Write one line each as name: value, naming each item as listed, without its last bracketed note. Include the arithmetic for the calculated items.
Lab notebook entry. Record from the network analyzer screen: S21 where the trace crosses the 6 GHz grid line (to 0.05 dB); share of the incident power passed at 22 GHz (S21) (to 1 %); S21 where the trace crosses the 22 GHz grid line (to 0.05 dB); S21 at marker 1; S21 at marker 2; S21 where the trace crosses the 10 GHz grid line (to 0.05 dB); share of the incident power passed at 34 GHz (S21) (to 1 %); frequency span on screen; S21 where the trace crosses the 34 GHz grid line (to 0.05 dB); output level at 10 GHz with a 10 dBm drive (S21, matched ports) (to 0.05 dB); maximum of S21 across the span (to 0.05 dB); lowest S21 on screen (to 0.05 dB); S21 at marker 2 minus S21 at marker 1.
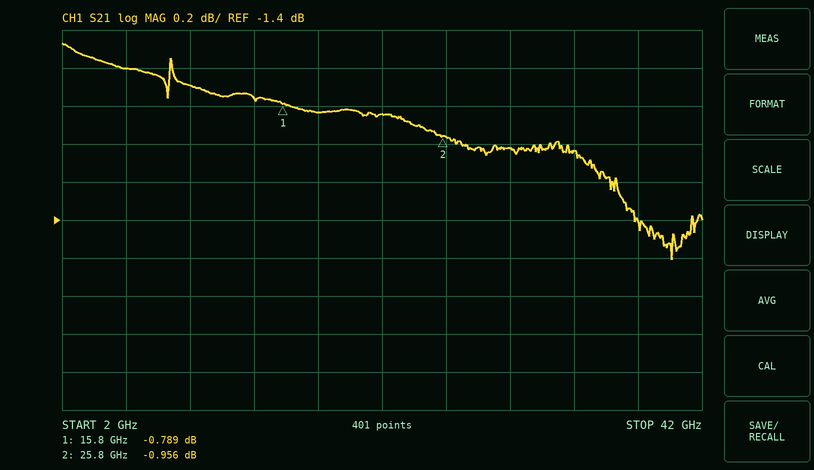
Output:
S21 where the trace crosses the 6 GHz grid line: -0.60 dB
share of the incident power passed at 22 GHz (S21): 10^(-0.85/10) ≈ 82 %
S21 where the trace crosses the 22 GHz grid line: -0.85 dB
S21 at marker 1: -0.789 dB
S21 at marker 2: -0.956 dB
S21 where the trace crosses the 10 GHz grid line: -0.70 dB
share of the incident power passed at 34 GHz (S21): 10^(-1.05/10) ≈ 79 %
frequency span on screen: 40 GHz
S21 where the trace crosses the 34 GHz grid line: -1.05 dB
output level at 10 GHz with a 10 dBm drive (S21, matched ports): 10 dBm + (-0.70 dB) = 9.30 dBm
maximum of S21 across the span: -0.45 dB
lowest S21 on screen: -1.60 dB
S21 at marker 2 minus S21 at marker 1: -0.956 − (-0.789) = -0.167 dB
